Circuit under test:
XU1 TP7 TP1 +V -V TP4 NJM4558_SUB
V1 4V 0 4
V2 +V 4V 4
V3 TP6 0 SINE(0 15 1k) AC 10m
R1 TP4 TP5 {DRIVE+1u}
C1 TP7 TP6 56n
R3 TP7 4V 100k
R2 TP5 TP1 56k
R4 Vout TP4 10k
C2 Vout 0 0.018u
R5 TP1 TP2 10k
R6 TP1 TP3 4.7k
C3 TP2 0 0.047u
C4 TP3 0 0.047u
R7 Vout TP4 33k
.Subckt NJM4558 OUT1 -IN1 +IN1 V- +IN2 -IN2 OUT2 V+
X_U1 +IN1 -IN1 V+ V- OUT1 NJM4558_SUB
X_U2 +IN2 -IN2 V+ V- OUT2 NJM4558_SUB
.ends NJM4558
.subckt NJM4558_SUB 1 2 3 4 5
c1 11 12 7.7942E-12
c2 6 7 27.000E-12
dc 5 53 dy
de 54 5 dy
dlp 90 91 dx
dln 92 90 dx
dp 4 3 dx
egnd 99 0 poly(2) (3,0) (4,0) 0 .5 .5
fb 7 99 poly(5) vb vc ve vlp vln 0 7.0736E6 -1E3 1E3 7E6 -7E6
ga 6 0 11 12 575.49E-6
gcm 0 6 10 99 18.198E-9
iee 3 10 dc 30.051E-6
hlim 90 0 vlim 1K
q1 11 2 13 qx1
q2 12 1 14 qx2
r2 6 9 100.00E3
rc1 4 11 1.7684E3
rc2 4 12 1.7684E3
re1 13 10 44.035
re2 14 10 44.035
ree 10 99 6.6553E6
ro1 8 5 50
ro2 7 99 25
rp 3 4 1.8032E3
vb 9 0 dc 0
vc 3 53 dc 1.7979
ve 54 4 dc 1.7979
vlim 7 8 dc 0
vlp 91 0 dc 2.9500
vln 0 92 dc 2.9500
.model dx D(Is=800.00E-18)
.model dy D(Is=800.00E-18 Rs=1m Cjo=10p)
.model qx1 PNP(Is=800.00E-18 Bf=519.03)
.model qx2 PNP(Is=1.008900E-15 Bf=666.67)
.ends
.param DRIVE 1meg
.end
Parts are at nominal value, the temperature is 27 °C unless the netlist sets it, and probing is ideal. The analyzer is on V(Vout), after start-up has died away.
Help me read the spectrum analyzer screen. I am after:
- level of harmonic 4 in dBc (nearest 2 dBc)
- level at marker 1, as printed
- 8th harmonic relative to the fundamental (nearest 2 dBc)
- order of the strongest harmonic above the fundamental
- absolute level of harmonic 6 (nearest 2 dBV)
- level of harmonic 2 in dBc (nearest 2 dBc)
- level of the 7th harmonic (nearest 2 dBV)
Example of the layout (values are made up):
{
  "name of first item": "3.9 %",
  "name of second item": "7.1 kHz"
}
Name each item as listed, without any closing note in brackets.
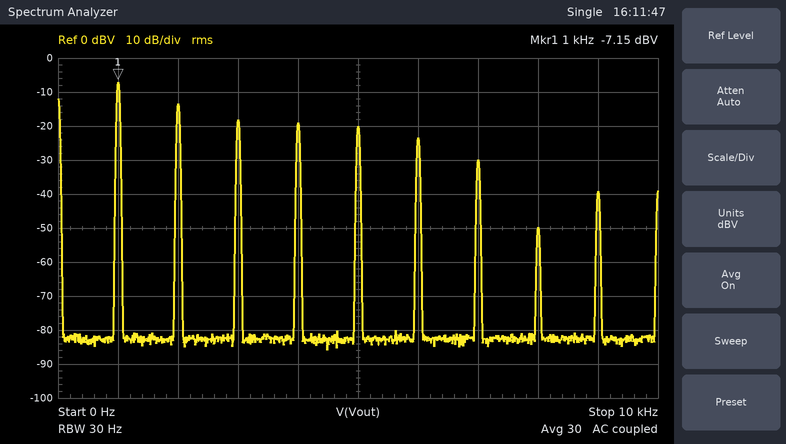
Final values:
{
  "level of harmonic 4 in dBc": "-12 dBc",
  "level at marker 1, as printed": "-7.15 dBV",
  "8th harmonic relative to the fundamental": "-42 dBc",
  "order of the strongest harmonic above the fundamental": "2",
  "absolute level of harmonic 6": "-24 dBV",
  "level of harmonic 2 in dBc": "-6 dBc",
  "level of the 7th harmonic": "-30 dBV"
}
